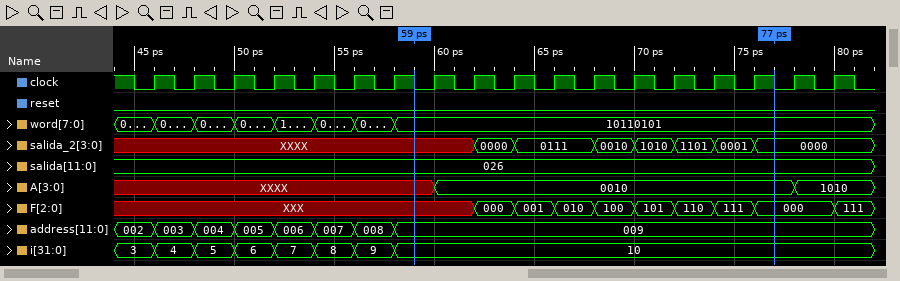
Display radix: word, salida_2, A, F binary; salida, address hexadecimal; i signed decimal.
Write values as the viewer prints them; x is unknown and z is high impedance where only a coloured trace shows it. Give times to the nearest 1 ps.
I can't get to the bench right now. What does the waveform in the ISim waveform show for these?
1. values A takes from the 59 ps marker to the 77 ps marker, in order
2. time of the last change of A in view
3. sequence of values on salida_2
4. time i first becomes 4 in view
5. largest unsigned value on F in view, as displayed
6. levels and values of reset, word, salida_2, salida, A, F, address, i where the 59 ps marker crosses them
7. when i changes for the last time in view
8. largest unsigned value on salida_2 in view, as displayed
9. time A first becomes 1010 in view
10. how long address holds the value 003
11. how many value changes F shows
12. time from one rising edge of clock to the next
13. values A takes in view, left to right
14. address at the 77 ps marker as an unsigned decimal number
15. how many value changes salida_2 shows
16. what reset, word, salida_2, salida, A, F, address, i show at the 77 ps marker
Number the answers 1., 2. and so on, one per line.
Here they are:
1. XXXX, 0010
2. 78 ps
3. XXXX, 0000, 0111, 0010, 1010, 1101, 0001, 0000
4. 46 ps
5. 111
6. reset=0, word=10110101, salida_2=XXXX, salida=026, A=XXXX, F=XXX, address=009, i=10
7. 58 ps
8. 1101
9. 78 ps
10. 2 ps
11. 9
12. 2 ps
13. XXXX, 0010, 1010
14. 9
15. 7
16. reset=0, word=10110101, salida_2=0000, salida=026, A=0010, F=000, address=009, i=10
